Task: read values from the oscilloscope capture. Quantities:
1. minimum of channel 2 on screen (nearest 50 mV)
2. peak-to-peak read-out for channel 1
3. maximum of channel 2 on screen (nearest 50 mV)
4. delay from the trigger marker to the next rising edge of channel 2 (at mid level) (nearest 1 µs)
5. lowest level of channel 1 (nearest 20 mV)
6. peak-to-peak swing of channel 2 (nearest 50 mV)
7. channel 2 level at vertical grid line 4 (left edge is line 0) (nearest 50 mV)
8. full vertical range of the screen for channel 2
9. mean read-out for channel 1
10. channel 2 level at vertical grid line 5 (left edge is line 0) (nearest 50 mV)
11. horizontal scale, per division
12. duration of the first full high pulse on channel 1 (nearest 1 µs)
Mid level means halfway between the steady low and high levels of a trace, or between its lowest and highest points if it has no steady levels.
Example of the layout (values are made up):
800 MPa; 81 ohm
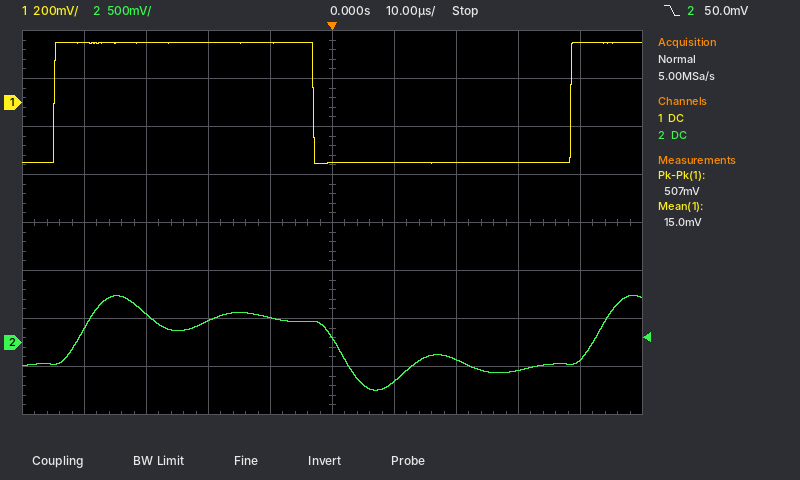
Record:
-500 mV; 507 mV; 500 mV; 42 µs; -260 mV; 1.00 V; 250 mV; 4 V; 15.0 mV; 50 mV; 10 µs; 42 µs
